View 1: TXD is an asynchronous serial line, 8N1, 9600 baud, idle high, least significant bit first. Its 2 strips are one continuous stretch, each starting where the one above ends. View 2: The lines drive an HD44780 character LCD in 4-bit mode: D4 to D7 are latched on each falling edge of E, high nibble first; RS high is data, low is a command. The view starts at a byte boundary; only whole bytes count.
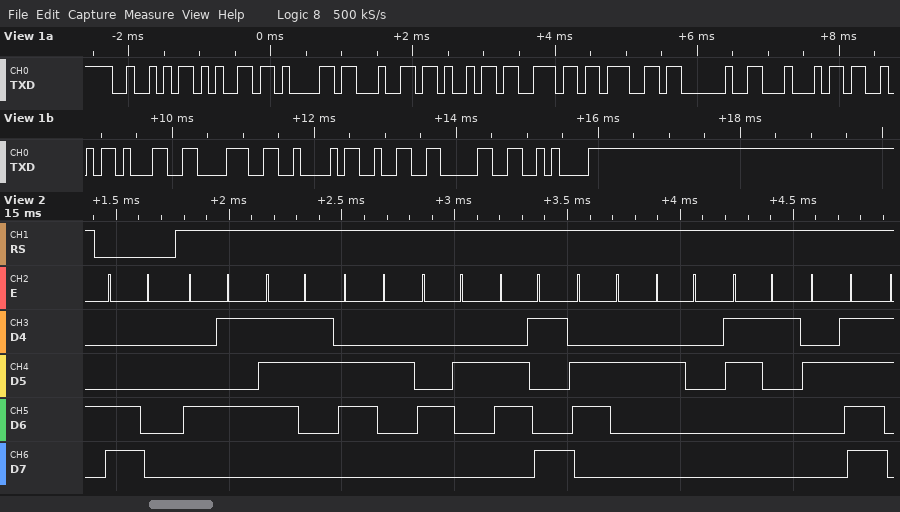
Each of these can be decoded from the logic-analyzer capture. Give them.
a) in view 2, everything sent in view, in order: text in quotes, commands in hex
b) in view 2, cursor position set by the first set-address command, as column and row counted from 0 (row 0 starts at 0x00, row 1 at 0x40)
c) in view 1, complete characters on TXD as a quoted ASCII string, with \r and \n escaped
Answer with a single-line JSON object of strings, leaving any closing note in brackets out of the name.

{"in view 2, everything sent in view, in order: text in quotes, commands in hex": "0xC0 \"EsbBib 1/\"", "in view 2, cursor position set by the first set-address command, as column and row counted from 0": "column 0, row 1", "in view 1, complete characters on TXD as a quoted ASCII string, with \\r and \\n escaped": "\"Reading DS18B20\\n\""}
